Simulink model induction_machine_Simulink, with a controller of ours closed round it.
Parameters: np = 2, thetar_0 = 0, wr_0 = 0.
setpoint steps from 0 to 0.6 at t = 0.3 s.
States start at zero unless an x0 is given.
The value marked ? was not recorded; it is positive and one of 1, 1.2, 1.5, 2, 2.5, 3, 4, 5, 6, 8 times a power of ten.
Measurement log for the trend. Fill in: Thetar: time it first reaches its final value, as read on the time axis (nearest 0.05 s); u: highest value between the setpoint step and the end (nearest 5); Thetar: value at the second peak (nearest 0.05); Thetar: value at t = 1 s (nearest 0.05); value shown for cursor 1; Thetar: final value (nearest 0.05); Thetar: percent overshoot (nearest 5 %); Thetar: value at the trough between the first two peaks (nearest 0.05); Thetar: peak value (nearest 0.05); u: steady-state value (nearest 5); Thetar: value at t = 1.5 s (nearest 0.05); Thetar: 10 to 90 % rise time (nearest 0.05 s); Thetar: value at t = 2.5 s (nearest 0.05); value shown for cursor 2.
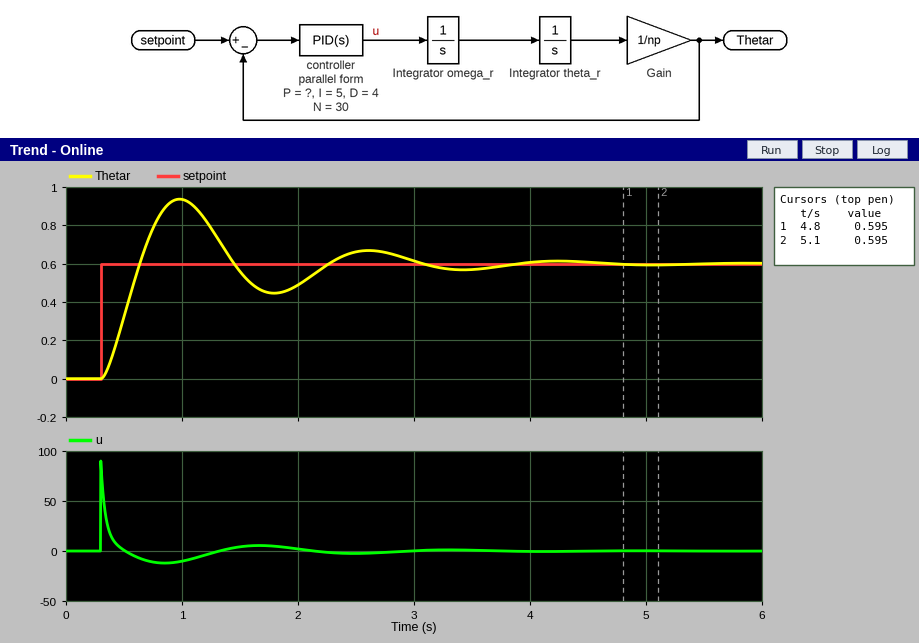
0.65 s
90
0.65
0.95
0.595
0.60
55 %
0.45
0.95
0
0.55
0.25 s
0.65
0.595
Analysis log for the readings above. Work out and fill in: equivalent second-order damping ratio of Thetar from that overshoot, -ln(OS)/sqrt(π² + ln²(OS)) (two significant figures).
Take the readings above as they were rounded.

0.19
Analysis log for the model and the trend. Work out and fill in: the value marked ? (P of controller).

30
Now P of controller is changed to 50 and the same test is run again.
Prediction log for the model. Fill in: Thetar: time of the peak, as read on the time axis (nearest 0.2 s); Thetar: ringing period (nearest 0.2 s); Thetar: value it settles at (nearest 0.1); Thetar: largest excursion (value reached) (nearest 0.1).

0.8 s
1.2 s
0.6
1.0
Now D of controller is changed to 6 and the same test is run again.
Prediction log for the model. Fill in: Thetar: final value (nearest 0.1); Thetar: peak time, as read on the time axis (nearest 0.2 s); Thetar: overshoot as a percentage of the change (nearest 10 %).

0.6
1.0 s
40 %
